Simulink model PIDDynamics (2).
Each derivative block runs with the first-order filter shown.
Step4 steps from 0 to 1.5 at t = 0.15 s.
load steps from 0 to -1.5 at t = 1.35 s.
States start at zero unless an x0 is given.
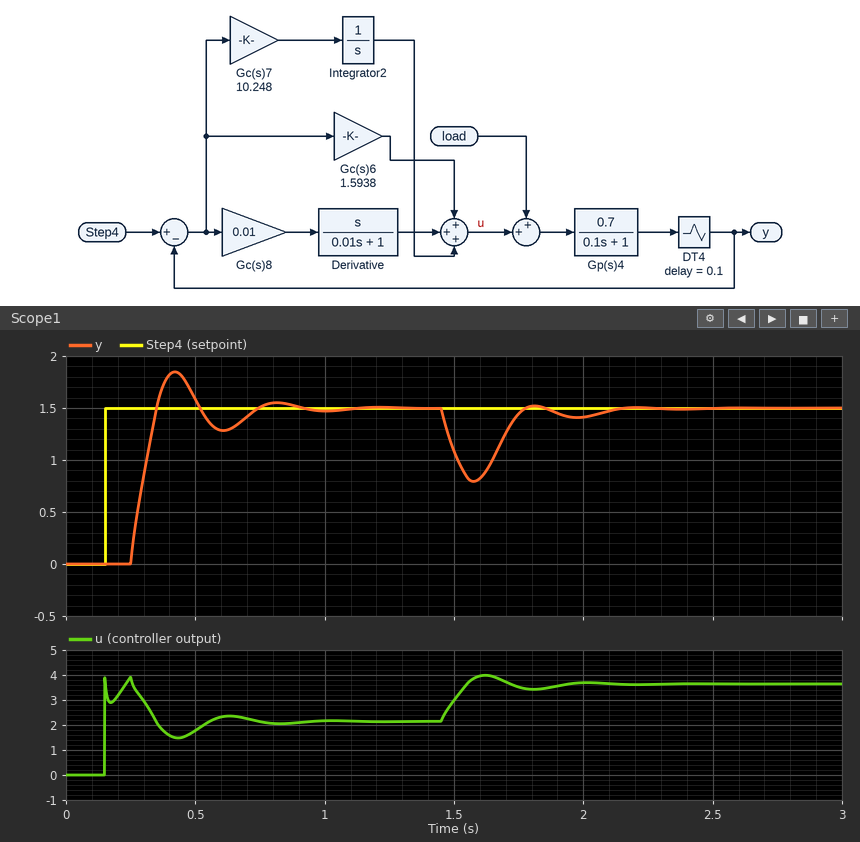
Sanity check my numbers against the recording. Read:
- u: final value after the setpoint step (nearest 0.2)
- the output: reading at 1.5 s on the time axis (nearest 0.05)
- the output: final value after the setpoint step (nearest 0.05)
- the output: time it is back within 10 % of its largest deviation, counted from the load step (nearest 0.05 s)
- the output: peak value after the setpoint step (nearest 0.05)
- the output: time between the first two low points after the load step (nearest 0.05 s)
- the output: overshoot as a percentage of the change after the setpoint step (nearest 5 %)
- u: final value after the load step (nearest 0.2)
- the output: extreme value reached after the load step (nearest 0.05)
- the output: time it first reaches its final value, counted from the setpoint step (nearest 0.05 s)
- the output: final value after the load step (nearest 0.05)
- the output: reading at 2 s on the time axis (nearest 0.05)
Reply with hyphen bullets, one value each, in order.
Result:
- 2.2
- 1.10
- 1.50
- 0.70 s
- 1.85
- 0.40 s
- 25 %
- 3.6
- 0.80
- 0.20 s
- 1.50
- 1.40
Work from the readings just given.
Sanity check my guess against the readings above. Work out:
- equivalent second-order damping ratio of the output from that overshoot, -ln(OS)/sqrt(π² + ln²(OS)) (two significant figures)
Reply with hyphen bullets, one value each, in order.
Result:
- 0.40
